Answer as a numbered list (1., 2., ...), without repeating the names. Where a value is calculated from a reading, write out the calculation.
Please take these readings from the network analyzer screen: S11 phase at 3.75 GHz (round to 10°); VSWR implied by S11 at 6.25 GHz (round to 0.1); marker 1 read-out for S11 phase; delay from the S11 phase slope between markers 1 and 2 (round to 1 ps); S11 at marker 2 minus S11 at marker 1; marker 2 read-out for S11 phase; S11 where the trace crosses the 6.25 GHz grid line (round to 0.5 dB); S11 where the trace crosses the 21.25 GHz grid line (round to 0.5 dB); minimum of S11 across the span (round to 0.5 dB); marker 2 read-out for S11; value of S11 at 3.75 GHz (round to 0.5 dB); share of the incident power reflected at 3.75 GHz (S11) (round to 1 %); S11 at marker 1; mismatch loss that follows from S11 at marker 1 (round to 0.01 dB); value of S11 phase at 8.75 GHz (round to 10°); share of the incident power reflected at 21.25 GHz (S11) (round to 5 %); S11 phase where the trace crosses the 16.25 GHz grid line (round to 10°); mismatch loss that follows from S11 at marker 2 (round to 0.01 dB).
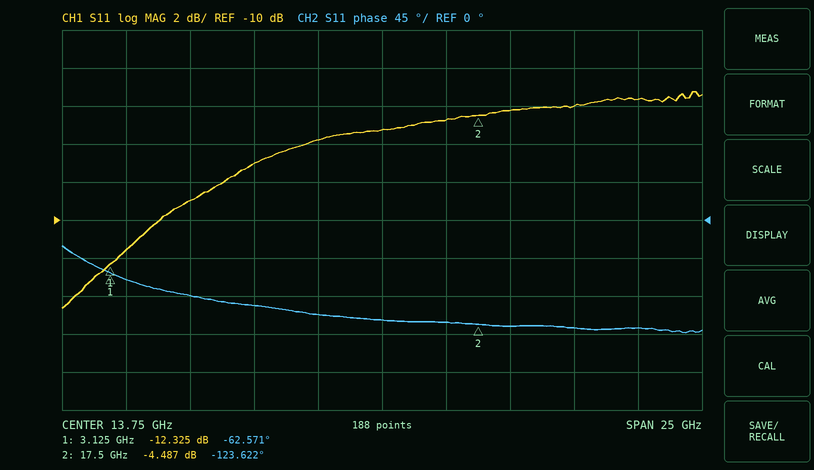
1. -70°
2. |Γ| = 10^(-9/20) = 0.3548; VSWR = (1 + 0.3548)/(1 − 0.3548) ≈ 2.1
3. -62.571°
4. −(-123.622° − (-62.571°))/(360° × 14.375 GHz) ≈ 12 ps
5. -4.487 − (-12.325) = 7.838 dB
6. -123.622°
7. -9.0 dB
8. -4.0 dB
9. -14.5 dB
10. -4.487 dB
11. -11.5 dB
12. 10^(-11.5/10) ≈ 7 %
13. -12.325 dB
14. −10 log10(1 − 10^(-12.325/10)) ≈ 0.26 dB
15. -100°
16. 10^(-4/10) ≈ 40 %
17. -120°
18. −10 log10(1 − 10^(-4.487/10)) ≈ 1.91 dB
